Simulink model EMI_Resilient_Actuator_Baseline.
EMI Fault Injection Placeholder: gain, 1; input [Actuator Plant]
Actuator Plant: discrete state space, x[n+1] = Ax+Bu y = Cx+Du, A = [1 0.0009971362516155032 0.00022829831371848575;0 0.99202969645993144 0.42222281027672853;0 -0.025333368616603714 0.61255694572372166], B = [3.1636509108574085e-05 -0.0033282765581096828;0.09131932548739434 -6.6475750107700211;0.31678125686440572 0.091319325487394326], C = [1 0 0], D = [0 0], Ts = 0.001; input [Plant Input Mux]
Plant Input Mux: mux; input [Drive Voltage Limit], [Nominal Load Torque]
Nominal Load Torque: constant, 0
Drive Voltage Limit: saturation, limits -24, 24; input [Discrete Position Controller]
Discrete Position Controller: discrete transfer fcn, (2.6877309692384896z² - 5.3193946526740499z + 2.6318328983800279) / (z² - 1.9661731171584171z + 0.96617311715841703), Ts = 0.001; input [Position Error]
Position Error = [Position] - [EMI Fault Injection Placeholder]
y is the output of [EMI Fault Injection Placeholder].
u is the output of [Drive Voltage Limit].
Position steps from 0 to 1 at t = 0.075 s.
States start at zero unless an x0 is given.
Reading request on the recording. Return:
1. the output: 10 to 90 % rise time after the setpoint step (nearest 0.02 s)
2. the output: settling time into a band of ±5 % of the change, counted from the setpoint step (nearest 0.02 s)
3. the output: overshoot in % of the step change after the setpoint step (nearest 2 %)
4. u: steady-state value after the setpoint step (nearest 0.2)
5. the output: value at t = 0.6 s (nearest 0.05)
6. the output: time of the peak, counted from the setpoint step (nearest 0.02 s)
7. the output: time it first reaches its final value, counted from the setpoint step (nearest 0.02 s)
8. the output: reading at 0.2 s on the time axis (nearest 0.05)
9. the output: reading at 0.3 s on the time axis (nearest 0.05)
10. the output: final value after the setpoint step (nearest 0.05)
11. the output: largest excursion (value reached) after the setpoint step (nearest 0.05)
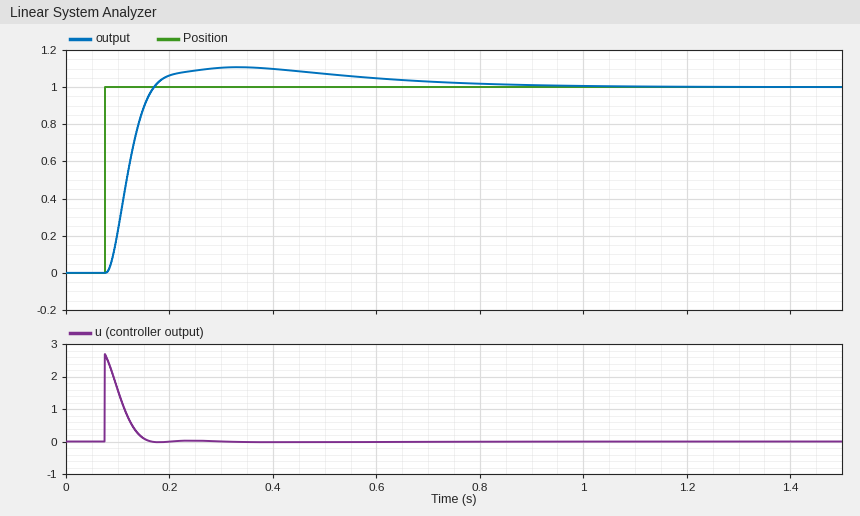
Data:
0.06 s
0.52 s
10 %
0.0
1.05
0.26 s
0.10 s
1.05
1.10
1.00
1.10
